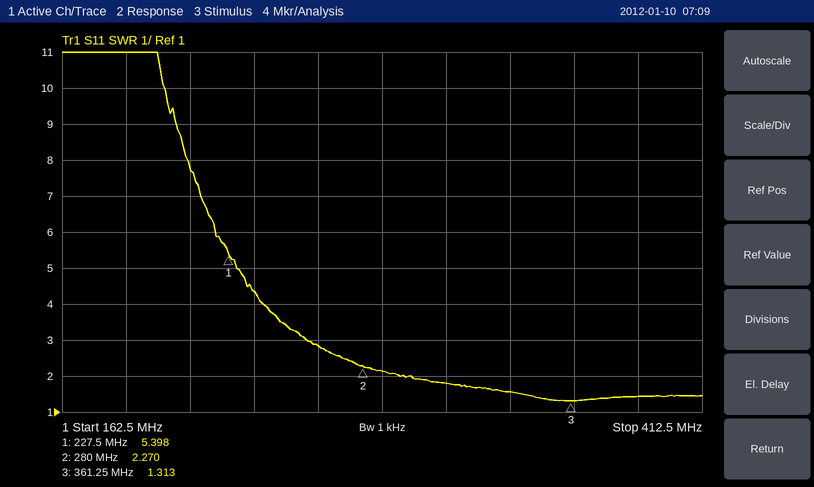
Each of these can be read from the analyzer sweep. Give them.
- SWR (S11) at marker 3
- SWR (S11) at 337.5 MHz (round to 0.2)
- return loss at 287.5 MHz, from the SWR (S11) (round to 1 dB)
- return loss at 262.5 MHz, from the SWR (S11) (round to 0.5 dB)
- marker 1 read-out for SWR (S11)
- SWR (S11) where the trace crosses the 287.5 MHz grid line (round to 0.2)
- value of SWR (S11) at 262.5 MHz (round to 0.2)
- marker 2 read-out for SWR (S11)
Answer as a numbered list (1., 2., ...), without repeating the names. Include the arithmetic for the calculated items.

1. 1.313
2. 1.6
3. −20 log10((2.2 − 1)/(2.2 + 1)) ≈ 9 dB
4. −20 log10((2.8 − 1)/(2.8 + 1)) ≈ 6.5 dB
5. 5.398
6. 2.2
7. 2.8
8. 2.270
